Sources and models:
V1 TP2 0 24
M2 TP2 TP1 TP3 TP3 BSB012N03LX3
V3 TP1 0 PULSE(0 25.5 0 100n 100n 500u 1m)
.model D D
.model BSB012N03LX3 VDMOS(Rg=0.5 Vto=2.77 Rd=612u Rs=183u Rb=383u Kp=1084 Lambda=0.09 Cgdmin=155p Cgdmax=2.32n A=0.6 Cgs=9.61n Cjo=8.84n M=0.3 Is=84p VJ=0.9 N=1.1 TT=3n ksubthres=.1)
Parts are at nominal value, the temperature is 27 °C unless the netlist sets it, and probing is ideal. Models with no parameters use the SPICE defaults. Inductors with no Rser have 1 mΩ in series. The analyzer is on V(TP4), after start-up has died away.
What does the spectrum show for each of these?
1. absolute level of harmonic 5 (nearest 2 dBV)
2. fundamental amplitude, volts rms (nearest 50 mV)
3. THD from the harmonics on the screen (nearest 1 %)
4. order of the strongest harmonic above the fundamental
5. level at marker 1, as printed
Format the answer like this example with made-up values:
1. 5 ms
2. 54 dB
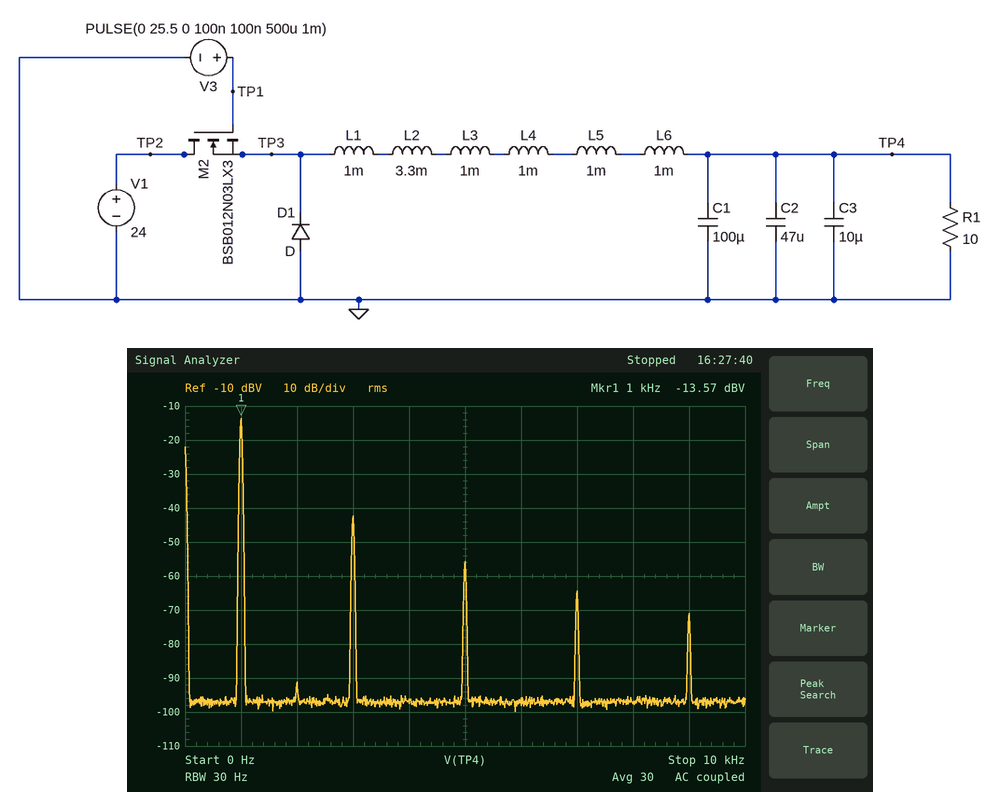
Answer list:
1. -56 dBV
2. 200 mV
3. 4 %
4. 3
5. -13.57 dBV
